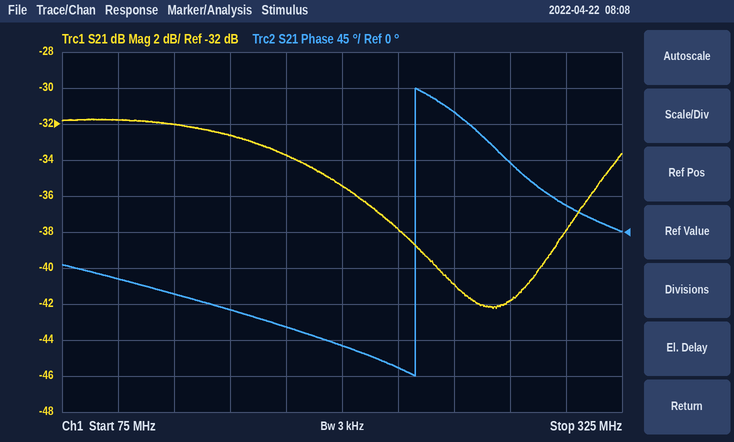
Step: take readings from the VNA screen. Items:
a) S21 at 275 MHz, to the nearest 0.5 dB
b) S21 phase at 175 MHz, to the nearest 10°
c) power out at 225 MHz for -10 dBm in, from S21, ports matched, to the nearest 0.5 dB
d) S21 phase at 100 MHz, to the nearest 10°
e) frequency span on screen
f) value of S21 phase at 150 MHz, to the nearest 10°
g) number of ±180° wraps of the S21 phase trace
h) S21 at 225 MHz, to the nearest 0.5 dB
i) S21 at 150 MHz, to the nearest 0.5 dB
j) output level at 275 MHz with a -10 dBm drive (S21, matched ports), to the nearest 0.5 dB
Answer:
-42.0 dB
-120°
-48.0 dBm
-60°
250 MHz
-100°
1
-38.0 dB
-32.5 dB
-52.0 dBm
